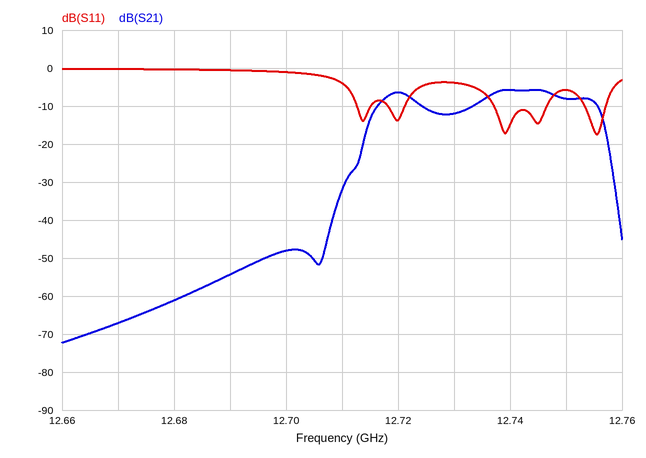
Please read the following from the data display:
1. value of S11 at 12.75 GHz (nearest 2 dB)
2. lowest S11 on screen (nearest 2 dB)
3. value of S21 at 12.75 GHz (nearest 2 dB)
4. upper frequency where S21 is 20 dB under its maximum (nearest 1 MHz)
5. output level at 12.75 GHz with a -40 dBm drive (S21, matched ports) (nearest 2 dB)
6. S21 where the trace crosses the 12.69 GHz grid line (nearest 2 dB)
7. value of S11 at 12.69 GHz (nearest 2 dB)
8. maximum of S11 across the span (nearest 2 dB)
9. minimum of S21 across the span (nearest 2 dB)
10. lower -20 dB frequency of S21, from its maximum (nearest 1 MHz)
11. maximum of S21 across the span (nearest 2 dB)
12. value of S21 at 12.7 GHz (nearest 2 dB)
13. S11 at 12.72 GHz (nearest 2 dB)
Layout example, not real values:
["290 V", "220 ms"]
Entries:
["-6 dB", "-18 dB", "-8 dB", "12.758 GHz", "-48 dBm", "-54 dB", "0 dB", "0 dB", "-72 dB", "12.713 GHz", "-6 dB", "-48 dB", "-14 dB"]
